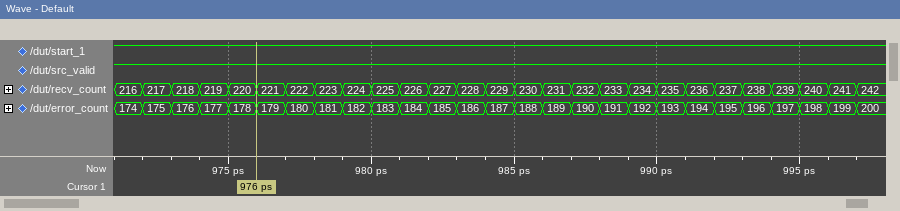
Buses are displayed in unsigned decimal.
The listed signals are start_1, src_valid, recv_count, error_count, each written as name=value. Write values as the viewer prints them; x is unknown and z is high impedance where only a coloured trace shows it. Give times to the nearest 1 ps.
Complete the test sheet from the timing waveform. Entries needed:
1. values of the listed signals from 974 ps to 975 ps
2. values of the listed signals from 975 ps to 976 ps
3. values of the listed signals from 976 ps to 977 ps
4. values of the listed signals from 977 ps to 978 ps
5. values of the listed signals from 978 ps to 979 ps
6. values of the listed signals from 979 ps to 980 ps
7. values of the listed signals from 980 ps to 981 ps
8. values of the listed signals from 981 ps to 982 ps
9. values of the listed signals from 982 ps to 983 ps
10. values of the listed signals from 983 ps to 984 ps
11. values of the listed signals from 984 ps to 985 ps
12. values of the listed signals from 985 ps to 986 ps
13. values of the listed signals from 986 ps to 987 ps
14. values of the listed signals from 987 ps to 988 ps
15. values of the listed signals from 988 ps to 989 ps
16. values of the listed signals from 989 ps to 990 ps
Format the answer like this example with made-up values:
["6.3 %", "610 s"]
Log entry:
["start_1=1, src_valid=1, recv_count=219, error_count=177", "start_1=1, src_valid=1, recv_count=220, error_count=178", "start_1=1, src_valid=1, recv_count=221, error_count=179", "start_1=1, src_valid=1, recv_count=222, error_count=180", "start_1=1, src_valid=1, recv_count=223, error_count=181", "start_1=1, src_valid=1, recv_count=224, error_count=182", "start_1=1, src_valid=1, recv_count=225, error_count=183", "start_1=1, src_valid=1, recv_count=226, error_count=184", "start_1=1, src_valid=1, recv_count=227, error_count=185", "start_1=1, src_valid=1, recv_count=228, error_count=186", "start_1=1, src_valid=1, recv_count=229, error_count=187", "start_1=1, src_valid=1, recv_count=230, error_count=188", "start_1=1, src_valid=1, recv_count=231, error_count=189", "start_1=1, src_valid=1, recv_count=232, error_count=190", "start_1=1, src_valid=1, recv_count=233, error_count=191", "start_1=1, src_valid=1, recv_count=234, error_count=192"]
